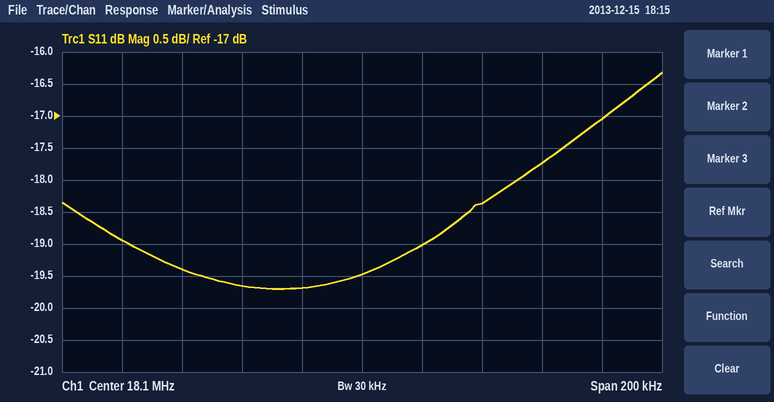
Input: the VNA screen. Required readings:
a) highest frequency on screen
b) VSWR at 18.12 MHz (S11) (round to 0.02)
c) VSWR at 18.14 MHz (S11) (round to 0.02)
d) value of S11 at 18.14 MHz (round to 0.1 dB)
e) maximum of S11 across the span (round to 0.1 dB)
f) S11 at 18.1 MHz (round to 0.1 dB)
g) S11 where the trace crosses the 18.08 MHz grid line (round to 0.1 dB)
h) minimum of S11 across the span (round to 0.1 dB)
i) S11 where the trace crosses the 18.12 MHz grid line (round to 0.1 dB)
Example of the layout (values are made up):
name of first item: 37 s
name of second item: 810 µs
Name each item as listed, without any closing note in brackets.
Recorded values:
highest frequency on screen: 18.2 MHz
VSWR at 18.12 MHz (S11): 1.26
VSWR at 18.14 MHz (S11): 1.28
value of S11 at 18.14 MHz: -18.4 dB
maximum of S11 across the span: -16.3 dB
S11 at 18.1 MHz: -19.5 dB
S11 where the trace crosses the 18.08 MHz grid line: -19.7 dB
minimum of S11 across the span: -19.7 dB
S11 where the trace crosses the 18.12 MHz grid line: -19.0 dB
